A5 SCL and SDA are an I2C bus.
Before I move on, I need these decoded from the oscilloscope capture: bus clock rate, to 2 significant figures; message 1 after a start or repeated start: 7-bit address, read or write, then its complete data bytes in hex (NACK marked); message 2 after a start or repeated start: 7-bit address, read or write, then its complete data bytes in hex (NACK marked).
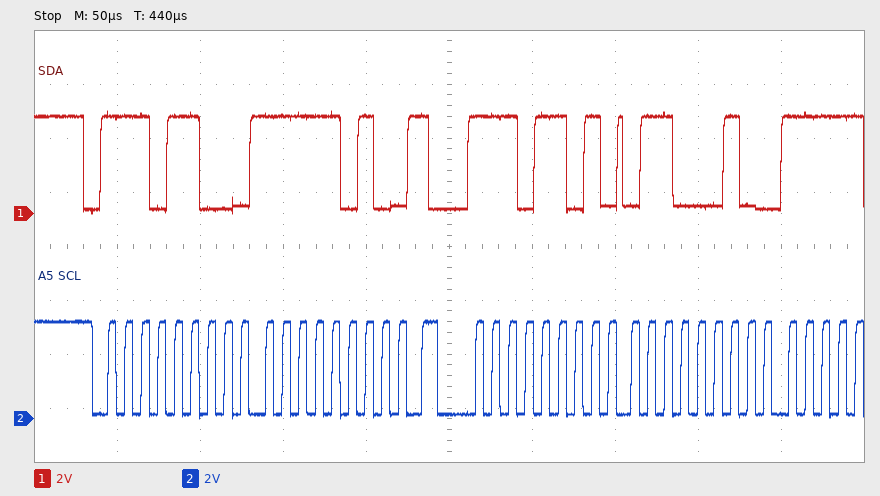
100 kHz
0x76 write: FA
0x76 read: 62
